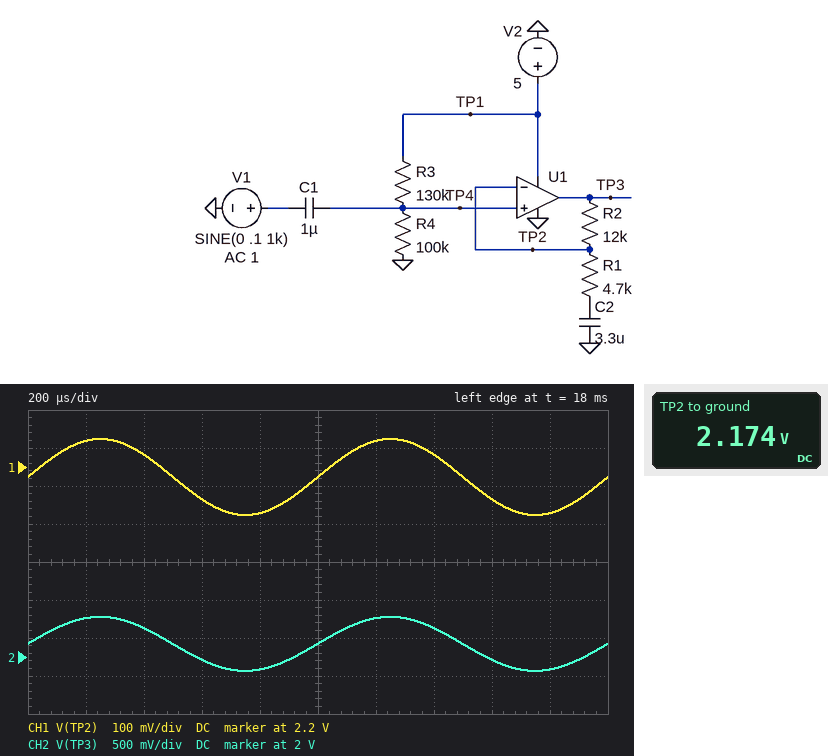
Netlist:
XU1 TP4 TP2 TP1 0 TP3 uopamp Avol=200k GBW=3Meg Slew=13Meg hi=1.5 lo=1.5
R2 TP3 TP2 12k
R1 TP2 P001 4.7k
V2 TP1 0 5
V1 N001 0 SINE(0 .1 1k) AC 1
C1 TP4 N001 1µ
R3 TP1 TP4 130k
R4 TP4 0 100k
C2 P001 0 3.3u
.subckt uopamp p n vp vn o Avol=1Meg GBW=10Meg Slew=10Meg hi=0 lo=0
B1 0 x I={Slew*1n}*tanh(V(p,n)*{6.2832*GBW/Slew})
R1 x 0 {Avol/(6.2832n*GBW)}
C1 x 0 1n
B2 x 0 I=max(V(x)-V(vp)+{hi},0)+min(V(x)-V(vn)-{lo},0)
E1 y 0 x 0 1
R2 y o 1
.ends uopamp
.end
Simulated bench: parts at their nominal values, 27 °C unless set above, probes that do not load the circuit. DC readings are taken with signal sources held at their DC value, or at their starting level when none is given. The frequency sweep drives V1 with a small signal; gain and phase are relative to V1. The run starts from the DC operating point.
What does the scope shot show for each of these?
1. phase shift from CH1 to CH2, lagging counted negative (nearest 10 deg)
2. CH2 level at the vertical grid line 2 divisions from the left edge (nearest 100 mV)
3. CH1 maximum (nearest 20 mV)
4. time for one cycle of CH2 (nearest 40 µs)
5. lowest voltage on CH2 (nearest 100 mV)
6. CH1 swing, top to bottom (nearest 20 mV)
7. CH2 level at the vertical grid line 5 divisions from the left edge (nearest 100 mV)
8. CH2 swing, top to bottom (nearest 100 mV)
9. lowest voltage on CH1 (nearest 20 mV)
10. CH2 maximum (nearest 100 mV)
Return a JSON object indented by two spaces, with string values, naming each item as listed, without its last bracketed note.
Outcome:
{
  "phase shift from CH1 to CH2, lagging counted negative": "0 deg",
  "CH2 level at the vertical grid line 2 divisions from the left edge": "2.4 V",
  "CH1 maximum": "2.28 V",
  "time for one cycle of CH2": "1.00 ms",
  "lowest voltage on CH2": "1.8 V",
  "CH1 swing, top to bottom": "200 mV",
  "CH2 level at the vertical grid line 5 divisions from the left edge": "2.2 V",
  "CH2 swing, top to bottom": "700 mV",
  "lowest voltage on CH1": "2.08 V",
  "CH2 maximum": "2.5 V"
}
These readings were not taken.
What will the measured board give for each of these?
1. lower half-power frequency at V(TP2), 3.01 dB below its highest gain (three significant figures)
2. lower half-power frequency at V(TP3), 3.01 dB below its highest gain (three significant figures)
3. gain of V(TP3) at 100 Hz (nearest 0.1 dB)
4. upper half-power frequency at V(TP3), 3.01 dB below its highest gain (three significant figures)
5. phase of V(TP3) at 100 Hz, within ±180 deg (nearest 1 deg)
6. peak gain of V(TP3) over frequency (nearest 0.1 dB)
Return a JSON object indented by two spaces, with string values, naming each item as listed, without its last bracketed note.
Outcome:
{
  "lower half-power frequency at V(TP2), 3.01 dB below its highest gain": "2.82 Hz",
  "lower half-power frequency at V(TP3), 3.01 dB below its highest gain": "10.2 Hz",
  "gain of V(TP3) at 100 Hz": "11.0 dB",
  "upper half-power frequency at V(TP3), 3.01 dB below its highest gain": "844 kHz",
  "phase of V(TP3) at 100 Hz, within ±180 deg": "6 deg",
  "peak gain of V(TP3) over frequency": "11.0 dB"
}
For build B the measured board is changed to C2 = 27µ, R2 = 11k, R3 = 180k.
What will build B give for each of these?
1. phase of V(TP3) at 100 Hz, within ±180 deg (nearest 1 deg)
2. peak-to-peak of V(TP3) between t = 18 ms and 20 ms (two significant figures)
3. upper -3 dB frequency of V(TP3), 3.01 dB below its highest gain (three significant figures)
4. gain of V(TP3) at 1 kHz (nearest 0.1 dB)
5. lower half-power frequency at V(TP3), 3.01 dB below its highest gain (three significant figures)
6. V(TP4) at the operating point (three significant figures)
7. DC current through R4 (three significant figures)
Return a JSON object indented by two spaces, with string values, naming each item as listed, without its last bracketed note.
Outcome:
{
  "phase of V(TP3) at 100 Hz, within ±180 deg": "2 deg",
  "peak-to-peak of V(TP3) between t = 18 ms and 20 ms": "620 mV",
  "upper -3 dB frequency of V(TP3), 3.01 dB below its highest gain": "898 kHz",
  "gain of V(TP3) at 1 kHz": "10.5 dB",
  "lower half-power frequency at V(TP3), 3.01 dB below its highest gain": "2.92 Hz",
  "V(TP4) at the operating point": "1.79 V",
  "DC current through R4": "17.9 µA"
}
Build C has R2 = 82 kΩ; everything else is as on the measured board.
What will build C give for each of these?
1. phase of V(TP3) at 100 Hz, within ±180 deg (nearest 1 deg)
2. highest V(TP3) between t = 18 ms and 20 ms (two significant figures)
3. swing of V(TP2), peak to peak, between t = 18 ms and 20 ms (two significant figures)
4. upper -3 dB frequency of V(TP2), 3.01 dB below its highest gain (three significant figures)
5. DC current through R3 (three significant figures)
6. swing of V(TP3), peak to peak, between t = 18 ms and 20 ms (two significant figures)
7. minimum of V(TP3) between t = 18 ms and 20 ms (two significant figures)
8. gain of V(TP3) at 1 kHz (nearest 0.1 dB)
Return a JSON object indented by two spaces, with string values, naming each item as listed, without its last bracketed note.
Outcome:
{
  "phase of V(TP3) at 100 Hz, within ±180 deg": "7 deg",
  "highest V(TP3) between t = 18 ms and 20 ms": "3.5 V",
  "swing of V(TP2), peak to peak, between t = 18 ms and 20 ms": "110 mV",
  "upper -3 dB frequency of V(TP2), 3.01 dB below its highest gain": "163 kHz",
  "DC current through R3": "21.7 µA",
  "swing of V(TP3), peak to peak, between t = 18 ms and 20 ms": "2.0 V",
  "minimum of V(TP3) between t = 18 ms and 20 ms": "1.5 V",
  "gain of V(TP3) at 1 kHz": "25.3 dB"
}
